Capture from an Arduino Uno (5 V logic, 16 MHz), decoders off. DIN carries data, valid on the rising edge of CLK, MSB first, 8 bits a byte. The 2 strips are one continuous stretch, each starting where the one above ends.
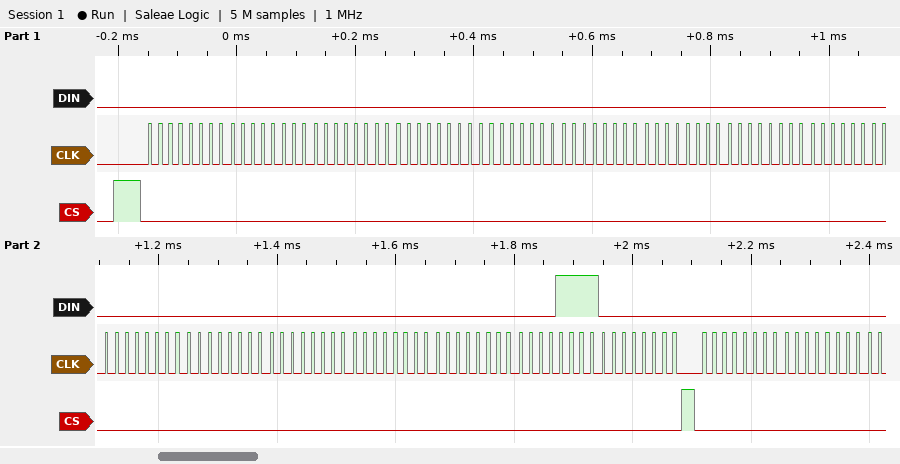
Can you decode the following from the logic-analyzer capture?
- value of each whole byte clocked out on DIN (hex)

0x00 0x00 0x00 0x00 0x00 0x00 0x00 0x00 0x00 0x00 0x00 0x00 0x00 0x00 0x0F 0x00 0x00 0x00
